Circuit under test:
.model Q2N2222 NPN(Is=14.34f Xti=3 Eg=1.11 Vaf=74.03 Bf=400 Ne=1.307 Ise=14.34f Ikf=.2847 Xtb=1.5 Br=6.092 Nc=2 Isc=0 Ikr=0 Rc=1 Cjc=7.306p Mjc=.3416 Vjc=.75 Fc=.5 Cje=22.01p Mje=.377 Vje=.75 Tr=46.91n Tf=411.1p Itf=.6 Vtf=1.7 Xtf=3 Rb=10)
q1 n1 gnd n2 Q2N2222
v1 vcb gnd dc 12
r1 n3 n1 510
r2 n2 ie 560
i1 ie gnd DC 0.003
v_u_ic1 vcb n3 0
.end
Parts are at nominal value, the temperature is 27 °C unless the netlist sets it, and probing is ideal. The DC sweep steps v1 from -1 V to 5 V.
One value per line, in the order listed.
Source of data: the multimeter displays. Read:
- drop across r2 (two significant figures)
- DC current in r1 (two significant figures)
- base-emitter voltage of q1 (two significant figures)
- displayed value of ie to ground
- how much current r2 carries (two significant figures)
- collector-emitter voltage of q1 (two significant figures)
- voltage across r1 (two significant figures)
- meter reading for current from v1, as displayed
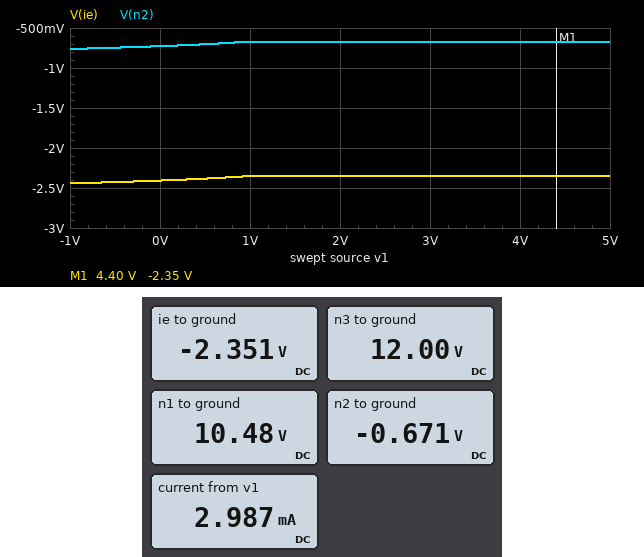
1.7 V
3.0 mA
670 mV
-2.351 V
3.0 mA
11 V
1.5 V
2.987 mA
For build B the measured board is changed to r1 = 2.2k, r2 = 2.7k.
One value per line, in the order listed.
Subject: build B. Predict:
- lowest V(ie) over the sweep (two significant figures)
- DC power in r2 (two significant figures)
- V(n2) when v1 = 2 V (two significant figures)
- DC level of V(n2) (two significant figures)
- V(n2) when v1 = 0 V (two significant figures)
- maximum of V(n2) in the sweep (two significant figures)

-8.9 V
24 mW
-730 mV
-670 mV
-750 mV
-690 mV
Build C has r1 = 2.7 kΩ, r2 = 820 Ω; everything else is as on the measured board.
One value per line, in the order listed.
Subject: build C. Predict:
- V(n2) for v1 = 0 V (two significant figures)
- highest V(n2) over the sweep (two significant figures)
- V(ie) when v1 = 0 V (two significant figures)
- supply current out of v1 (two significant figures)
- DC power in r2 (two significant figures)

-750 mV
-710 mV
-3.2 V
3.0 mA
7.4 mW
